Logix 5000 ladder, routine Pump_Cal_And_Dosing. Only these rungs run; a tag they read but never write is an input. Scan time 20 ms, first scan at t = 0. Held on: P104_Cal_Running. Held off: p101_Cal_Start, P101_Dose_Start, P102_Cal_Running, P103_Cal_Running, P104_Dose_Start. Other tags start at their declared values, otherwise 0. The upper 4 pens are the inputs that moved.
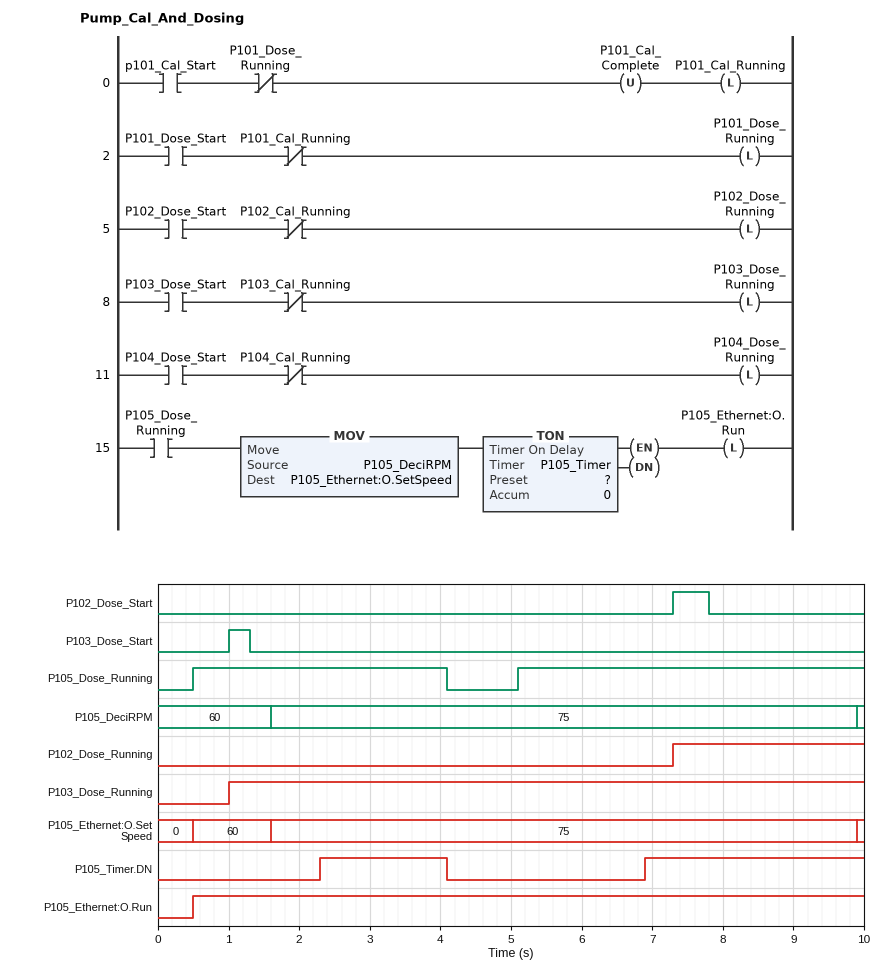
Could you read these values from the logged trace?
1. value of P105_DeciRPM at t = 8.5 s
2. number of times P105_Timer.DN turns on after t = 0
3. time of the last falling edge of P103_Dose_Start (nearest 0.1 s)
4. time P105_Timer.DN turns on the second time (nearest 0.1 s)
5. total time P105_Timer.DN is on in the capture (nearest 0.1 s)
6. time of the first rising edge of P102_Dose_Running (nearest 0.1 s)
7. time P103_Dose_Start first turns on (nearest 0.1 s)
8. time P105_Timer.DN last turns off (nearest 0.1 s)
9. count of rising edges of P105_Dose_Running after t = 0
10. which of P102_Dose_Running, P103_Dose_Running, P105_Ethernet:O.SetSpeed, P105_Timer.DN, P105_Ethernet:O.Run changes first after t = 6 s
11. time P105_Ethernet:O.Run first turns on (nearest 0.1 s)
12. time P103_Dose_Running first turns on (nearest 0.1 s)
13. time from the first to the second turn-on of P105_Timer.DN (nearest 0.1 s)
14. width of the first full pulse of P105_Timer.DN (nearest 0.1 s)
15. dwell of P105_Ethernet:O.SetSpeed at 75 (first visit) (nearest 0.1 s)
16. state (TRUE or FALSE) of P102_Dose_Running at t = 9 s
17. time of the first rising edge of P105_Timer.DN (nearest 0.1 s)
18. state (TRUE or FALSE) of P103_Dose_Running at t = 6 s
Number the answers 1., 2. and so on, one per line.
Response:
1. 75
2. 2
3. 1.3 s
4. 6.9 s
5. 4.9 s
6. 7.3 s
7. 1.0 s
8. 4.1 s
9. 2
10. P105_Timer.DN
11. 0.5 s
12. 1.0 s
13. 4.6 s
14. 1.8 s
15. 8.3 s
16. TRUE
17. 2.3 s
18. TRUE
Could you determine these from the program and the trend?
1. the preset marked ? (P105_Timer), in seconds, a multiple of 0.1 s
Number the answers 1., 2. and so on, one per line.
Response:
1. 1.8 s
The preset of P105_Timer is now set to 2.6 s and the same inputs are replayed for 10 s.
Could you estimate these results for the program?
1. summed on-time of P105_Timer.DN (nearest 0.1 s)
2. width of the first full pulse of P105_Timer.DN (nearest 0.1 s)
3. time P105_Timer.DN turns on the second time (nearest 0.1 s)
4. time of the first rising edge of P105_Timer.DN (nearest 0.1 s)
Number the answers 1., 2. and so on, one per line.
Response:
1. 3.3 s
2. 1.0 s
3. 7.7 s
4. 3.1 s
